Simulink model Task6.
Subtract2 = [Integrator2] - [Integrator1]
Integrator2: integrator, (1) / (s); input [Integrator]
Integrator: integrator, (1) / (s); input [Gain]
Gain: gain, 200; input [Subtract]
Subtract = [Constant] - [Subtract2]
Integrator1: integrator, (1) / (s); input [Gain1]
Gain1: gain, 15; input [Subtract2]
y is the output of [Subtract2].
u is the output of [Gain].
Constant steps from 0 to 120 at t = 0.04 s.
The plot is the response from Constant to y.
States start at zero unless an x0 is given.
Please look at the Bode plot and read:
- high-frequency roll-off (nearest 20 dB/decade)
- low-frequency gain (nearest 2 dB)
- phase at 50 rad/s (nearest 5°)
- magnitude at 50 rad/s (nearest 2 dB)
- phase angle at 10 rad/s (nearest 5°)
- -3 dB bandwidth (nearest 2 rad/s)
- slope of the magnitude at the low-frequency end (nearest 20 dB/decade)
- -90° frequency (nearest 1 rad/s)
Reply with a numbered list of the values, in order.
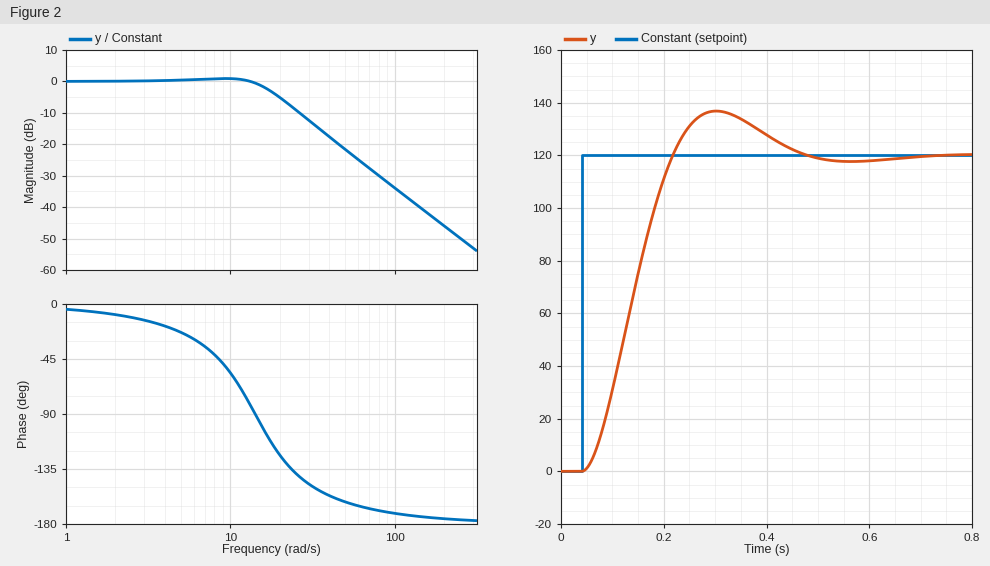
1. -40 dB/decade
2. 0 dB
3. -160°
4. -22 dB
5. -55°
6. 18 rad/s
7. 0 dB/decade
8. 14 rad/s
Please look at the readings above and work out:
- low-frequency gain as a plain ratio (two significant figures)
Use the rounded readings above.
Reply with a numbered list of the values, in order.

1. 1.0
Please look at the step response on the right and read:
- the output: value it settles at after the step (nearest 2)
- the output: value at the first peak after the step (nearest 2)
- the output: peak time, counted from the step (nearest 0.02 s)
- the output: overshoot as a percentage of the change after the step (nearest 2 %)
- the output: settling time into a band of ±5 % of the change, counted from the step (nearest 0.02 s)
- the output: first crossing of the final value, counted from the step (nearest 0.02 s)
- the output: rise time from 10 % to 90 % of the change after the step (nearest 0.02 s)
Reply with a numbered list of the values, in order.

1. 120
2. 136
3. 0.26 s
4. 14 %
5. 0.38 s
6. 0.18 s
7. 0.12 s
